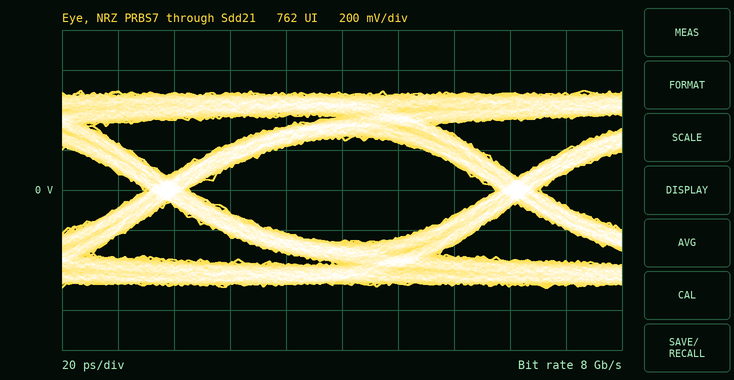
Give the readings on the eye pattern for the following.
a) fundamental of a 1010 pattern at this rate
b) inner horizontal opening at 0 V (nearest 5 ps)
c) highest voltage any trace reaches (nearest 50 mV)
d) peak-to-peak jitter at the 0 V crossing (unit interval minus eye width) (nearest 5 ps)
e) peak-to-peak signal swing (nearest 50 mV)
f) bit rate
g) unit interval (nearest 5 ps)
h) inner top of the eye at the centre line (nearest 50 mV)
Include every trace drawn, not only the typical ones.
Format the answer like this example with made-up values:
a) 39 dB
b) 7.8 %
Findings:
a) 4 GHz
b) 110 ps
c) 500 mV
d) 15 ps
e) 1.00 V
f) 8 Gb/s
g) 125 ps
h) 250 mV
